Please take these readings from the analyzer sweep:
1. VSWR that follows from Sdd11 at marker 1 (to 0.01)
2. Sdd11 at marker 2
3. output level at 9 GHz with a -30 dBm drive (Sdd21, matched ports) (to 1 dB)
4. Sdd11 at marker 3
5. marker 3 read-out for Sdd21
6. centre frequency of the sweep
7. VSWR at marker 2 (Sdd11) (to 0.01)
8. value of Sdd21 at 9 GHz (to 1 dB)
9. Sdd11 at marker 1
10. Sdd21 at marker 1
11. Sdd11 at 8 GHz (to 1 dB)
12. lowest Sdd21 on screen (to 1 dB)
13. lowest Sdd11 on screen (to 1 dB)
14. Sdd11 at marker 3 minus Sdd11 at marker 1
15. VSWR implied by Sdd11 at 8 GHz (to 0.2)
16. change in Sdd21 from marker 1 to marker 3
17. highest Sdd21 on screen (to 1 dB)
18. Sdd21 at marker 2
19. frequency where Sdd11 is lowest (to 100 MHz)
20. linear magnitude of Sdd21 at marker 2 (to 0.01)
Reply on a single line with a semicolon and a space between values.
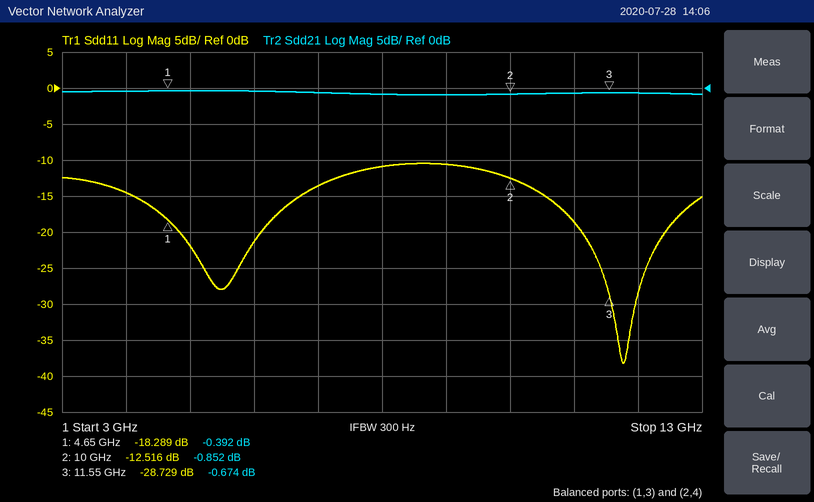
1.28; -12.516 dB; -31 dBm; -28.729 dB; -0.674 dB; 8 GHz; 1.62; -1 dB; -18.289 dB; -0.392 dB; -11 dB; -1 dB; -38 dB; -10.440 dB; 1.8; -0.282 dB; 0 dB; -0.852 dB; 11.8 GHz; 0.91
